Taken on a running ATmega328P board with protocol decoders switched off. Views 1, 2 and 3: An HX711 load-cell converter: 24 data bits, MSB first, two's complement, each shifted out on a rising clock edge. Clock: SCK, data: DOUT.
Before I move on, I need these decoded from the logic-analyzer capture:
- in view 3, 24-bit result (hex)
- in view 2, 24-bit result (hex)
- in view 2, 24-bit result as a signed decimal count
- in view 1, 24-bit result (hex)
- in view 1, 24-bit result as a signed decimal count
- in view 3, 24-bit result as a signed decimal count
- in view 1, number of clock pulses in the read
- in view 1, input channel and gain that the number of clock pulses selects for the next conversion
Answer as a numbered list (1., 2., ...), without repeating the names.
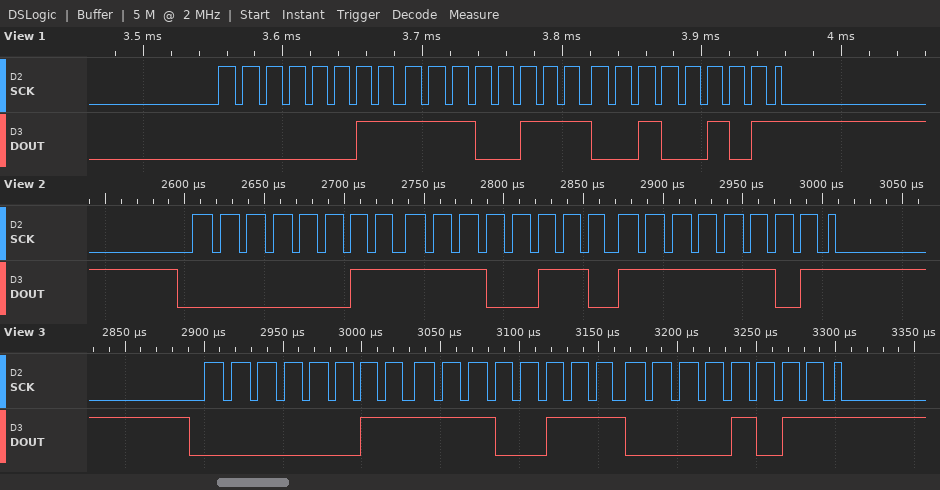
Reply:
1. 0x03E70B
2. 0x03E6FD
3. 255741
4. 0x03E725
5. 255781
6. 255755
7. 25
8. channel A, gain 128
